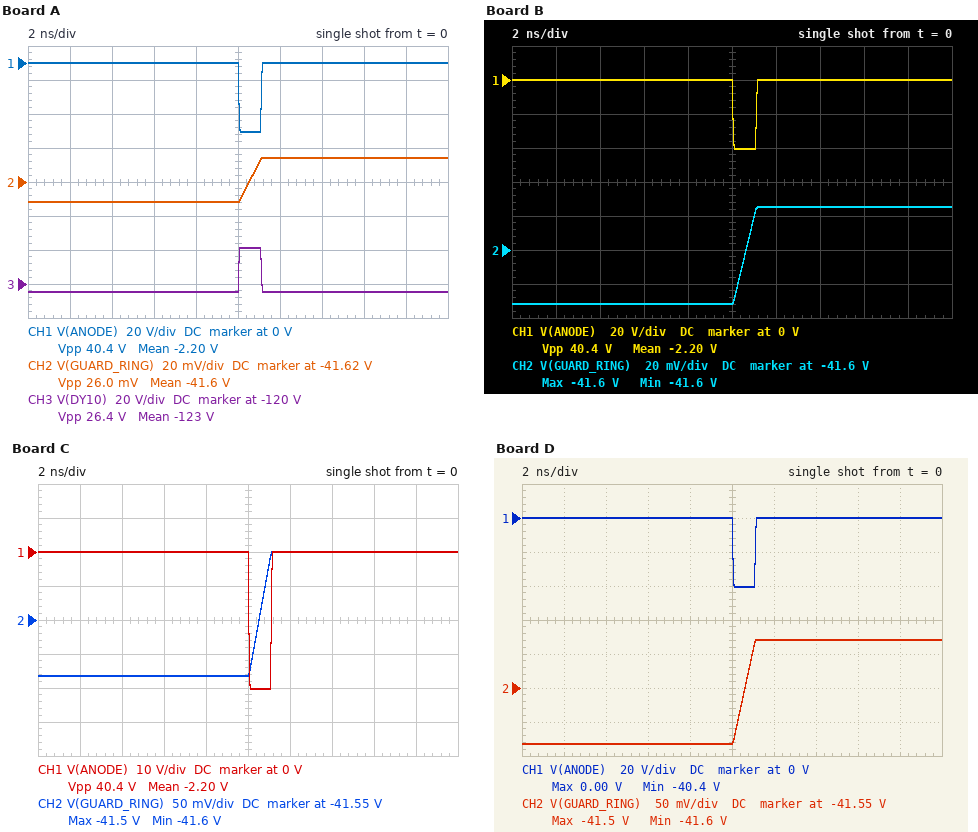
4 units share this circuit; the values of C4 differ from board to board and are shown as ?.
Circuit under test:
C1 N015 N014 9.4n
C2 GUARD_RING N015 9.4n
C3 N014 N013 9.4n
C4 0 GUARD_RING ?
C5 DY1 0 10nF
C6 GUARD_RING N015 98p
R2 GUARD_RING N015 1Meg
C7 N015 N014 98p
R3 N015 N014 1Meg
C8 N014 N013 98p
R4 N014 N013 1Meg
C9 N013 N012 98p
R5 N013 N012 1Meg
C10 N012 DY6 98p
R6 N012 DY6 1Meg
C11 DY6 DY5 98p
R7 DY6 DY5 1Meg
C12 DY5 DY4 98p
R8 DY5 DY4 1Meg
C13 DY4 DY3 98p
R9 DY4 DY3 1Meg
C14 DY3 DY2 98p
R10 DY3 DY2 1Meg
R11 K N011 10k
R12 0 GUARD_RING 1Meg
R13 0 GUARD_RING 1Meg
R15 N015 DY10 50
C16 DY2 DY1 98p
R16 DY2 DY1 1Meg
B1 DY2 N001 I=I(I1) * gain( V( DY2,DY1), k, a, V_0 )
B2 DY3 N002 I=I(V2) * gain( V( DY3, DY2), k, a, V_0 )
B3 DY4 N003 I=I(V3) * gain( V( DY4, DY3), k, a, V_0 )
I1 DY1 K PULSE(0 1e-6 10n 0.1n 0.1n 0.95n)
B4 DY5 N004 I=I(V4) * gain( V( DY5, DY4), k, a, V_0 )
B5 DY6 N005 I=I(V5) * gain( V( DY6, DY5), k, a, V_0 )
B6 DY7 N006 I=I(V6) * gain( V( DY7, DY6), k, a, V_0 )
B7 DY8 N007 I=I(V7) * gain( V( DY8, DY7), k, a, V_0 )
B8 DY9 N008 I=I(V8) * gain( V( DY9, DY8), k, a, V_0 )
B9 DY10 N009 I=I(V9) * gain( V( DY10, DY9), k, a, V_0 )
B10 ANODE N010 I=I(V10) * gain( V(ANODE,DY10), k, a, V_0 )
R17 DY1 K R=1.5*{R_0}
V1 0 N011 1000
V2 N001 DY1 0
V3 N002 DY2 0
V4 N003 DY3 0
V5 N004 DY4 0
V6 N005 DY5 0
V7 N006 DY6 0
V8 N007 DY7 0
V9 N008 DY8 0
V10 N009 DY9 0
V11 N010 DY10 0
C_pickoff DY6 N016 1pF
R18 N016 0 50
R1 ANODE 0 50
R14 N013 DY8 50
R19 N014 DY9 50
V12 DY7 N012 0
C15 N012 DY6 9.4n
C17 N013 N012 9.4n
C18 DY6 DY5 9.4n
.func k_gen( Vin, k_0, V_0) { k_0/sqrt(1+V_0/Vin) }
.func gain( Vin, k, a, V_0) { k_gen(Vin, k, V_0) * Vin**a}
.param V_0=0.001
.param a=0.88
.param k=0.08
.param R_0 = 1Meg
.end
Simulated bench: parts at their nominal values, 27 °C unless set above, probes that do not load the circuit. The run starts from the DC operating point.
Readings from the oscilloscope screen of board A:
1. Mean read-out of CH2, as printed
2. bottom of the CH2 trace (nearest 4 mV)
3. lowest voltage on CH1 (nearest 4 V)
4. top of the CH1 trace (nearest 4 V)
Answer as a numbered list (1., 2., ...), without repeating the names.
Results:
1. -41.6 V
2. -41.632 V
3. -40 V
4. 0 V
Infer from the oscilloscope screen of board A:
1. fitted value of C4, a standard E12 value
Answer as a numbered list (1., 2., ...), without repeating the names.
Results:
1. 33 nF
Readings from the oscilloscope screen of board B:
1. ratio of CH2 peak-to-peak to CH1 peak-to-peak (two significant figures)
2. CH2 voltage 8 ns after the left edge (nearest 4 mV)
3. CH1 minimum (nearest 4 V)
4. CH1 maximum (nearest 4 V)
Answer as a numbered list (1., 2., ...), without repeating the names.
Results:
1. 0.0014
2. -41.632 V
3. -40 V
4. 0 V
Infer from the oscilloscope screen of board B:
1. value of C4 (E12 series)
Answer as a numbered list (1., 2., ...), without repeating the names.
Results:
1. 15 nF
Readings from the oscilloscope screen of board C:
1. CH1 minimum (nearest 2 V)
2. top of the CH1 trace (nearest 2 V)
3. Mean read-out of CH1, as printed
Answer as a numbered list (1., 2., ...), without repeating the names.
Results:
1. -40 V
2. 0 V
3. -2.20 V
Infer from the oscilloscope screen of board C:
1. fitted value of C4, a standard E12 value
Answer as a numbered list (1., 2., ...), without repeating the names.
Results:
1. 4.7 nF
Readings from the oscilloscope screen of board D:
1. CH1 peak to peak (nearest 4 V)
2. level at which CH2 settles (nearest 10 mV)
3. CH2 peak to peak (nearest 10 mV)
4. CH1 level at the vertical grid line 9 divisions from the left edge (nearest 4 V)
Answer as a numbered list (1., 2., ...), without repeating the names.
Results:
1. 40 V
2. -41.48 V
3. 150 mV
4. 0 V
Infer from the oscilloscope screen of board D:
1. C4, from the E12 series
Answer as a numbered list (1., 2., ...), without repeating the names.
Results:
1. 5.6 nF
